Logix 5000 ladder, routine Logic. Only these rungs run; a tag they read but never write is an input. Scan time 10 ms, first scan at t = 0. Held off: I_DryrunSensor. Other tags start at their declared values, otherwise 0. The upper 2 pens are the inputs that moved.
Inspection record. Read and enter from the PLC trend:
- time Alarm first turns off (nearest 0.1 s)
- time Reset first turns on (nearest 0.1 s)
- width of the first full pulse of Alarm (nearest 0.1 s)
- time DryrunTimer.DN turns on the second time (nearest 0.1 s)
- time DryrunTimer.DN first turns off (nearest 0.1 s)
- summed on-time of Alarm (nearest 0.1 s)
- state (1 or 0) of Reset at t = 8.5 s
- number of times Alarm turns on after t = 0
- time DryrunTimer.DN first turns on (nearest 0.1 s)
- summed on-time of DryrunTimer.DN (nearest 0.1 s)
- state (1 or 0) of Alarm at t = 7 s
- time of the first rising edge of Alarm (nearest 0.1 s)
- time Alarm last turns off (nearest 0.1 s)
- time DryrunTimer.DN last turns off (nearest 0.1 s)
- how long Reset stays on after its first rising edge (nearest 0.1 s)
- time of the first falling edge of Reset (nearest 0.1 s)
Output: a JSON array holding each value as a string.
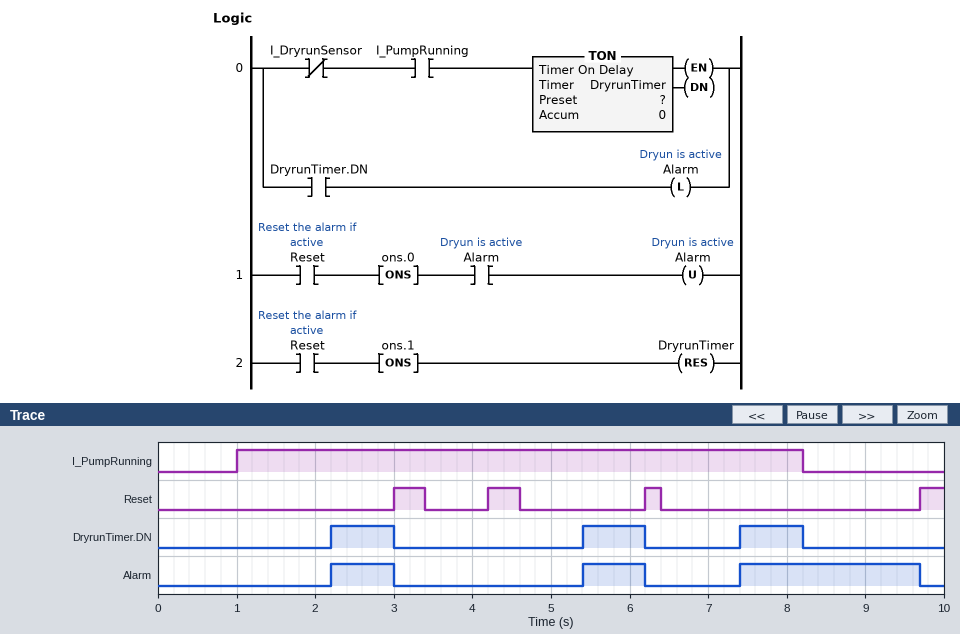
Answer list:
["3.0 s", "3.0 s", "0.8 s", "5.4 s", "3.0 s", "3.9 s", "0", "3", "2.2 s", "2.4 s", "0", "2.2 s", "9.7 s", "8.2 s", "0.4 s", "3.4 s"]
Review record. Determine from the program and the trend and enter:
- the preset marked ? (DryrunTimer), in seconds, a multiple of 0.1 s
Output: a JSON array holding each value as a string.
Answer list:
["1.2 s"]
